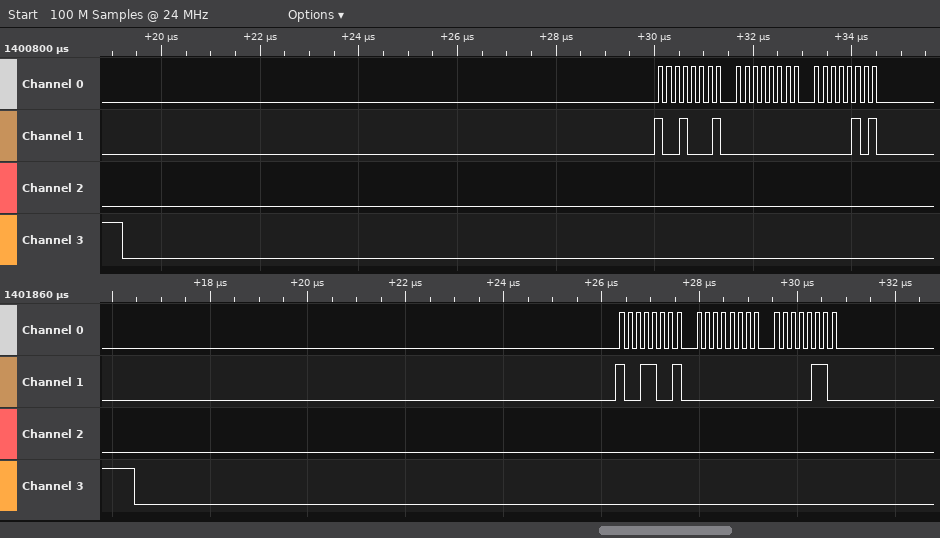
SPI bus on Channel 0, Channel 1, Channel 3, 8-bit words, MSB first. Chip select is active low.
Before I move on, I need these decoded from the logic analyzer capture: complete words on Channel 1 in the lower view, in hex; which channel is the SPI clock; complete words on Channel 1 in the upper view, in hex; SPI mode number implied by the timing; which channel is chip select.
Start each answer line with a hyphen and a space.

- 99, 00, 06
- Channel 0
- 91, 00, 05
- 0
- Channel 3
